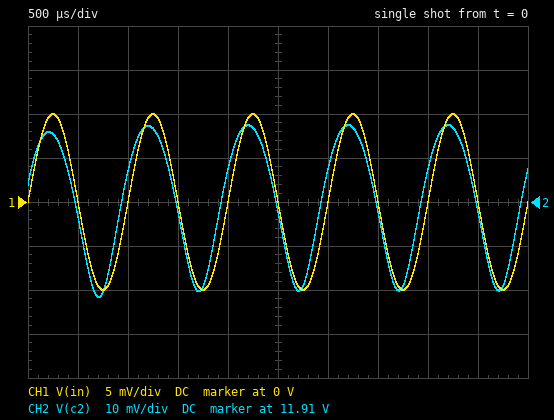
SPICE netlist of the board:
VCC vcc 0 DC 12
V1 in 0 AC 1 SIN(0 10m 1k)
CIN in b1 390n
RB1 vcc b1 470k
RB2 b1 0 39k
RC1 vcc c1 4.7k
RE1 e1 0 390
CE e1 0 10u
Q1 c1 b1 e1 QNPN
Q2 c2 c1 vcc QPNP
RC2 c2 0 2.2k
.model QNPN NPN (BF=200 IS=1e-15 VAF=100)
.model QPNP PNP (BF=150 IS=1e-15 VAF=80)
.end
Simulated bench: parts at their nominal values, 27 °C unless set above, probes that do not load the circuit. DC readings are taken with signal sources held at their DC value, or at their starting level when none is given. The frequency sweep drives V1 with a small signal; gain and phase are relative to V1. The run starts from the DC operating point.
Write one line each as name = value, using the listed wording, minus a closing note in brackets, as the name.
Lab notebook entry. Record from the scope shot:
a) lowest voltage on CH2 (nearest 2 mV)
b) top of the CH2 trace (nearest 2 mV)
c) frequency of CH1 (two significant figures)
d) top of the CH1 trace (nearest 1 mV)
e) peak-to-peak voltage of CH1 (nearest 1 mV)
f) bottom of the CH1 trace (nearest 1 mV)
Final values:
lowest voltage on CH2 = 11.888 V
top of the CH2 trace = 11.928 V
frequency of CH1 = 1.0 kHz
top of the CH1 trace = 10 mV
peak-to-peak voltage of CH1 = 20 mV
bottom of the CH1 trace = -10 mV
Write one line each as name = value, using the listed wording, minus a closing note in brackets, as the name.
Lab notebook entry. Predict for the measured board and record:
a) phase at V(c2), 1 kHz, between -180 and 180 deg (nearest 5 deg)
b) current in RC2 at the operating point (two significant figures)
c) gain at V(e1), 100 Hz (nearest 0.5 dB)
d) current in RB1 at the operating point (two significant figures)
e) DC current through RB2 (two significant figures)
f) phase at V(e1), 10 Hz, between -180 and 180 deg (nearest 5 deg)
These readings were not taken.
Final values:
phase at V(c2), 1 kHz, between -180 and 180 deg = 15 deg
current in RC2 at the operating point = 5.4 mA
gain at V(e1), 100 Hz = -2.5 dB
current in RB1 at the operating point = 24 µA
DC current through RB2 = 22 µA
phase at V(e1), 10 Hz, between -180 and 180 deg = 55 deg
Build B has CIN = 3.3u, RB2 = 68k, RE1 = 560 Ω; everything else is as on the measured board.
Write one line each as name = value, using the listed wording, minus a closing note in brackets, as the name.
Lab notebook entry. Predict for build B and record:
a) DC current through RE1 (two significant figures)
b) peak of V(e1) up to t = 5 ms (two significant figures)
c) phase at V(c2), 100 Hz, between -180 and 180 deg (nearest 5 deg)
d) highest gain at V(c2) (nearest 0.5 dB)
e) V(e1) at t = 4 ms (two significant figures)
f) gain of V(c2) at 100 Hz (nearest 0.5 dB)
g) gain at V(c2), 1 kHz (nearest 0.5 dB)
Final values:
DC current through RE1 = 970 µA
peak of V(e1) up to t = 5 ms = 550 mV
phase at V(c2), 100 Hz, between -180 and 180 deg = 65 deg
highest gain at V(c2) = 0 dB
V(e1) at t = 4 ms = 540 mV
gain of V(c2) at 100 Hz = -16.0 dB
gain at V(c2), 1 kHz = -1.5 dB
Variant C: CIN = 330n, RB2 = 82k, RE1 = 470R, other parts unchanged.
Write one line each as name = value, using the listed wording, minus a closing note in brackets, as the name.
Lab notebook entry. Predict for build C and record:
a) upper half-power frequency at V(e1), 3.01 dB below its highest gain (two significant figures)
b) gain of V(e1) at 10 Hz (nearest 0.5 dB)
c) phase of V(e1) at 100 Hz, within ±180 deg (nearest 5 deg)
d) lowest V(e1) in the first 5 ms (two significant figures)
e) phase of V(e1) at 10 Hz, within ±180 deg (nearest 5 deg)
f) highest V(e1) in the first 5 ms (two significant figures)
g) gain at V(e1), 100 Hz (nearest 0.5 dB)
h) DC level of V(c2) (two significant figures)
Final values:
upper half-power frequency at V(e1), 3.01 dB below its highest gain = 1.0 kHz
gain of V(e1) at 10 Hz = -4.5 dB
phase of V(e1) at 100 Hz, within ±180 deg = 0 deg
lowest V(e1) in the first 5 ms = 630 mV
phase of V(e1) at 10 Hz, within ±180 deg = 45 deg
highest V(e1) in the first 5 ms = 640 mV
gain at V(e1), 100 Hz = -1.5 dB
DC level of V(c2) = 12 V
